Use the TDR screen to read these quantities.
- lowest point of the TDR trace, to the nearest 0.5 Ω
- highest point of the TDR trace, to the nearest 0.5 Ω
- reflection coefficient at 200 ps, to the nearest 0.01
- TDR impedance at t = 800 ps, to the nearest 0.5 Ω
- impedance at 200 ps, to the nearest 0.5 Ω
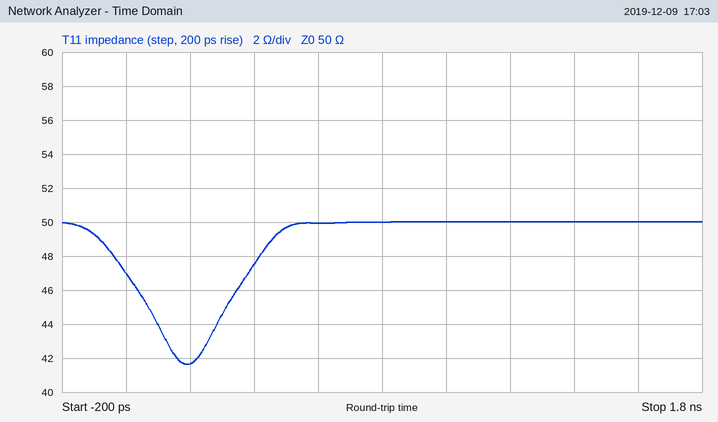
41.5 Ω
50.0 Ω
-0.09
50.0 Ω
41.5 Ω
